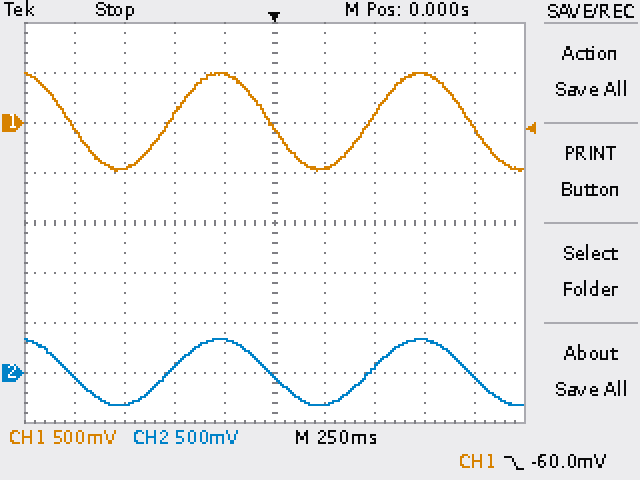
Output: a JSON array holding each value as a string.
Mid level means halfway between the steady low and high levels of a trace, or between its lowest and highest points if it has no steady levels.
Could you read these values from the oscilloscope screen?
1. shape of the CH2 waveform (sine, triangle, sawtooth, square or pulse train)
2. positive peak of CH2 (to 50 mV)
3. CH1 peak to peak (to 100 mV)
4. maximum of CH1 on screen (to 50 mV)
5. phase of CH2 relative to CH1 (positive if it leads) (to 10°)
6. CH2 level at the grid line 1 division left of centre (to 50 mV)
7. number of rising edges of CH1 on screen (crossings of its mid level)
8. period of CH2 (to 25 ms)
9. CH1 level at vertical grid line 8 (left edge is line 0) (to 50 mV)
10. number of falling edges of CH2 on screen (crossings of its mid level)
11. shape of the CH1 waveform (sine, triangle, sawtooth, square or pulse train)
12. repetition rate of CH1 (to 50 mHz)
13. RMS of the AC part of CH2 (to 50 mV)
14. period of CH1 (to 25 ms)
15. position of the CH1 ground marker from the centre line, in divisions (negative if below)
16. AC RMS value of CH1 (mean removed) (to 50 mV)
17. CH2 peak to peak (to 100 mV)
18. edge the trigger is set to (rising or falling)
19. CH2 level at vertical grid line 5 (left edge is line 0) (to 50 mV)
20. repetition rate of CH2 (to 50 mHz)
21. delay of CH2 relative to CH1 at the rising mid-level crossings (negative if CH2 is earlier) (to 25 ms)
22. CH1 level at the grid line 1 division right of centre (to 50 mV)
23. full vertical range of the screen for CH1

["sine", "350 mV", "1.00 V", "500 mV", "0°", "350 mV", "2", "1.000 s", "500 mV", "3", "sine", "1.00 Hz", "250 mV", "1.000 s", "+2.0 div", "350 mV", "700 mV", "falling", "-50 mV", "1.00 Hz", "0 ms", "-450 mV", "4 V"]
